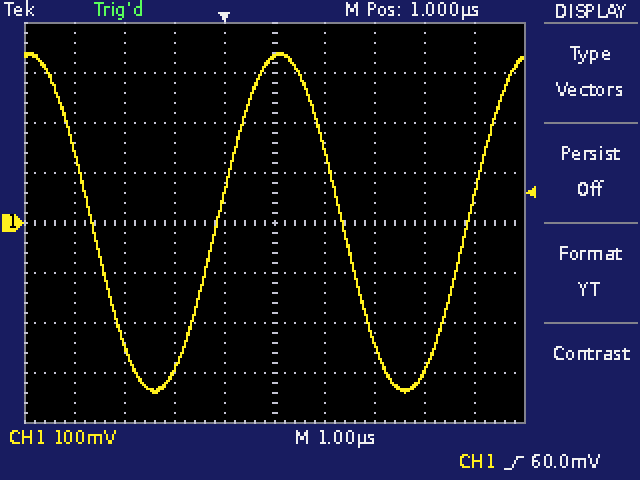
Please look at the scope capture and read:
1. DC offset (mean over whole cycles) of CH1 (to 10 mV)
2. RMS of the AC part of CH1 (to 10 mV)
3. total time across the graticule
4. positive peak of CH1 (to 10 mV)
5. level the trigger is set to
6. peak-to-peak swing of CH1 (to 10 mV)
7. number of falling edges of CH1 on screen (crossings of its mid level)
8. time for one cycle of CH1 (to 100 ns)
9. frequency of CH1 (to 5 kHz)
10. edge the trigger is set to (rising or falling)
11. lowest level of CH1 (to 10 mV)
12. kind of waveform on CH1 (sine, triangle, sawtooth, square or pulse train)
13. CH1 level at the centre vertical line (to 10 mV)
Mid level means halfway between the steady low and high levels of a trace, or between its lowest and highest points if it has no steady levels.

0 mV
240 mV
10 µs
340 mV
60.0 mV
680 mV
2
5.0 µs
200 kHz
rising
-340 mV
sine
330 mV
